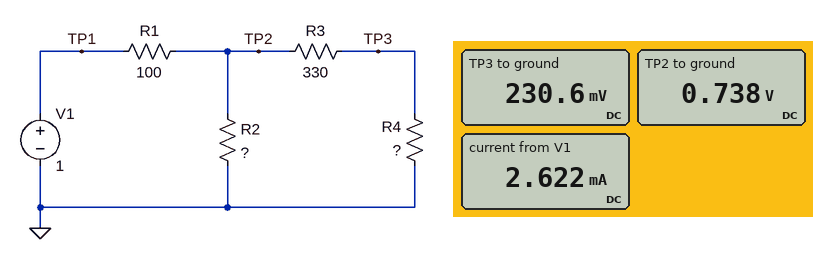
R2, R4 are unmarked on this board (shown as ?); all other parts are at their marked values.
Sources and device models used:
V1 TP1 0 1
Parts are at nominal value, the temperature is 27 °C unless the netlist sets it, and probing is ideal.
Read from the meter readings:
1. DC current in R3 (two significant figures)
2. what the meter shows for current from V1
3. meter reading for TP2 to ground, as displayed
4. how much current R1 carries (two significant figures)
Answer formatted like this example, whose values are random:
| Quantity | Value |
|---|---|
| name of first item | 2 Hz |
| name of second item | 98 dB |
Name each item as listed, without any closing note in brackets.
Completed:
| Quantity | Value |
|---|---|
| DC current in R3 | 1.5 mA |
| what the meter shows for current from V1 | 2.622 mA |
| meter reading for TP2 to ground, as displayed | 0.738 V |
| how much current R1 carries | 2.6 mA |
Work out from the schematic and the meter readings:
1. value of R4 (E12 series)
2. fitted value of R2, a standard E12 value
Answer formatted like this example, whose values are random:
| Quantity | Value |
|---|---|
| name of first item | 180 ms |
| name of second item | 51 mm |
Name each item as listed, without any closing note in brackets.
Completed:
| Quantity | Value |
|---|---|
| value of R4 | 150 Ω |
| fitted value of R2, a standard E12 value | 680 Ω |
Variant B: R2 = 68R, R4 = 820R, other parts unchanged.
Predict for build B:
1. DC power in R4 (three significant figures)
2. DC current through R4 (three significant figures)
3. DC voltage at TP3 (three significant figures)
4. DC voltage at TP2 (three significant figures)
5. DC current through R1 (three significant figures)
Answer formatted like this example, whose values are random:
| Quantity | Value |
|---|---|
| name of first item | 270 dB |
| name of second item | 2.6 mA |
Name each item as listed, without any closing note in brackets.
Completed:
| Quantity | Value |
|---|---|
| DC power in R4 | 94.8 µW |
| DC current through R4 | 340 µA |
| DC voltage at TP3 | 279 mV |
| DC voltage at TP2 | 391 mV |
| DC current through R1 | 6.09 mA |
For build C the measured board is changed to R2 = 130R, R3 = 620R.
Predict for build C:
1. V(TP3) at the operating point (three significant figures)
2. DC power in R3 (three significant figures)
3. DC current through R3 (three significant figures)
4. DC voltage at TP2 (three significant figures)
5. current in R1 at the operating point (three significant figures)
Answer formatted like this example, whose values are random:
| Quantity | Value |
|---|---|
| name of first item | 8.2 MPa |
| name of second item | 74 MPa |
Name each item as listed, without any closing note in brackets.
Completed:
| Quantity | Value |
|---|---|
| V(TP3) at the operating point | 103 mV |
| DC power in R3 | 290 µW |
| DC current through R3 | 684 µA |
| DC voltage at TP2 | 527 mV |
| current in R1 at the operating point | 4.73 mA |
